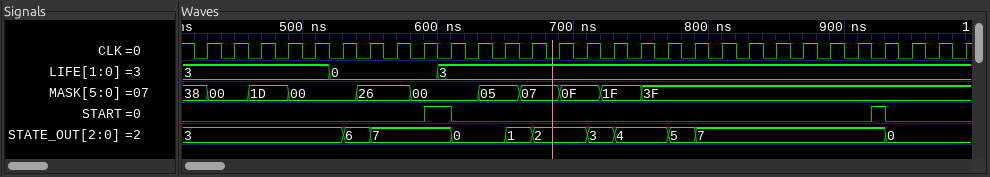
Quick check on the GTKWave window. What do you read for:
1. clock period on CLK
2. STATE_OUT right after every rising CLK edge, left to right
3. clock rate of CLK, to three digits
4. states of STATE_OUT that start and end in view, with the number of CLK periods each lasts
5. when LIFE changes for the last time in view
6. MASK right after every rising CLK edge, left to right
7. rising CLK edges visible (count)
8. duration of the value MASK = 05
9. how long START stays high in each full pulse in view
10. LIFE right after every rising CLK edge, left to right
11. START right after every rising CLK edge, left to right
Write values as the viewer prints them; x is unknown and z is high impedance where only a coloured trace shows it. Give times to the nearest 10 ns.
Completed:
20 ns
3, 3, 3, 3, 3, 6, 7, 7, 7, 0, 0, 1, 2, 2, 3, 4, 4, 5, 7, 7, 7, 7, 7, 7, 7, 0, 0, 0, 0
50.0 MHz
6: 1, 7: 3, 0: 2, 1: 1, 2: 2, 3: 1, 4: 2, 5: 1, 7: 7
600 ns
00, 00, 1D, 00, 00, 00, 26, 26, 00, 00, 05, 05, 07, 0F, 0F, 1F, 3F, 3F, 3F, 3F, 3F, 3F, 3F, 3F, 3F, 3F, 3F, 3F, 3F
29
30 ns
20 ns, 10 ns
3, 3, 3, 3, 3, 0, 0, 0, 0, 3, 3, 3, 3, 3, 3, 3, 3, 3, 3, 3, 3, 3, 3, 3, 3, 3, 3, 3, 3
0 0 0 0 0 0 0 0 1 0 0 0 0 0 0 0 0 0 0 0 0 0 0 0 0 0 0 0 0
